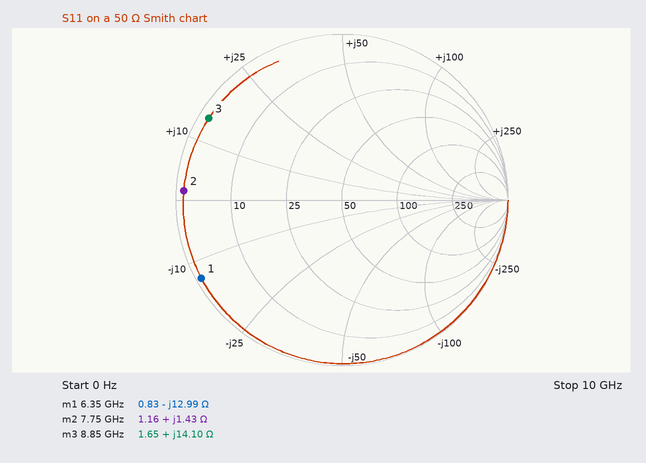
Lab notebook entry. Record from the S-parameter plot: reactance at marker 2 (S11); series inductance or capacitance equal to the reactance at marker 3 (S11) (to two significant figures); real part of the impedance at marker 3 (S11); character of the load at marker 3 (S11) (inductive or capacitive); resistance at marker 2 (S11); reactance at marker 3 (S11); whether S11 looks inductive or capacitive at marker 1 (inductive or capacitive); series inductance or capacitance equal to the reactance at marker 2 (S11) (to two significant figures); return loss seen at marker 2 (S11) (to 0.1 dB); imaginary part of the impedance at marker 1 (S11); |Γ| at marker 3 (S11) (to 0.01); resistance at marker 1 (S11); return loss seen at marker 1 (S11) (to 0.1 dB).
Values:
+1.43 Ω
250 pH
1.65 Ω
inductive
1.16 Ω
+14.10 Ω
capacitive
29 pH
0.4 dB
-12.99 Ω
0.94
0.83 Ω
0.3 dB
